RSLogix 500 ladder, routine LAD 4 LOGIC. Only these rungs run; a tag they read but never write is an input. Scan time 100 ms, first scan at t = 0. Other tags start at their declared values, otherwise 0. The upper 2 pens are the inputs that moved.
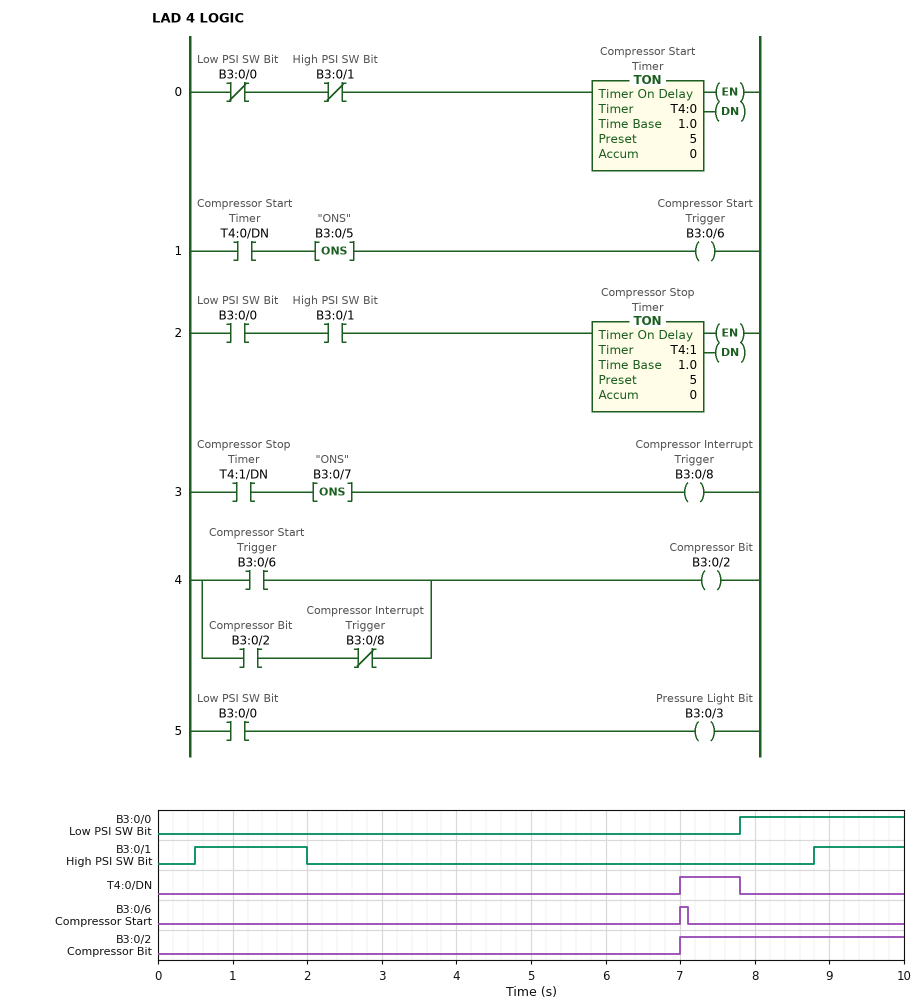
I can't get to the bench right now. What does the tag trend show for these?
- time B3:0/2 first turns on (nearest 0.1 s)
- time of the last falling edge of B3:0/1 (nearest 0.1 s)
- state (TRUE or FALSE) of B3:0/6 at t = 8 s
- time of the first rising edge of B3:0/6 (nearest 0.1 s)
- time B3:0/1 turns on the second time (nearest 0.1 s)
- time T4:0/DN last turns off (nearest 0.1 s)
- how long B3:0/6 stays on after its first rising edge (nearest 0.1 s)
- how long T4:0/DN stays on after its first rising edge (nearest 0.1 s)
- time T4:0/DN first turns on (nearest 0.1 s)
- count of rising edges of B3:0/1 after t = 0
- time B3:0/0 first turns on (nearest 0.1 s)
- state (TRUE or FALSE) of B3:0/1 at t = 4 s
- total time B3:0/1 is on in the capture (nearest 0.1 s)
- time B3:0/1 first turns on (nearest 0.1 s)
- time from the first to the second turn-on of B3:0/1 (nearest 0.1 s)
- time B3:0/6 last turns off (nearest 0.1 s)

7.0 s
2.0 s
FALSE
7.0 s
8.8 s
7.8 s
0.1 s
0.8 s
7.0 s
2
7.8 s
FALSE
2.7 s
0.5 s
8.3 s
7.1 s
